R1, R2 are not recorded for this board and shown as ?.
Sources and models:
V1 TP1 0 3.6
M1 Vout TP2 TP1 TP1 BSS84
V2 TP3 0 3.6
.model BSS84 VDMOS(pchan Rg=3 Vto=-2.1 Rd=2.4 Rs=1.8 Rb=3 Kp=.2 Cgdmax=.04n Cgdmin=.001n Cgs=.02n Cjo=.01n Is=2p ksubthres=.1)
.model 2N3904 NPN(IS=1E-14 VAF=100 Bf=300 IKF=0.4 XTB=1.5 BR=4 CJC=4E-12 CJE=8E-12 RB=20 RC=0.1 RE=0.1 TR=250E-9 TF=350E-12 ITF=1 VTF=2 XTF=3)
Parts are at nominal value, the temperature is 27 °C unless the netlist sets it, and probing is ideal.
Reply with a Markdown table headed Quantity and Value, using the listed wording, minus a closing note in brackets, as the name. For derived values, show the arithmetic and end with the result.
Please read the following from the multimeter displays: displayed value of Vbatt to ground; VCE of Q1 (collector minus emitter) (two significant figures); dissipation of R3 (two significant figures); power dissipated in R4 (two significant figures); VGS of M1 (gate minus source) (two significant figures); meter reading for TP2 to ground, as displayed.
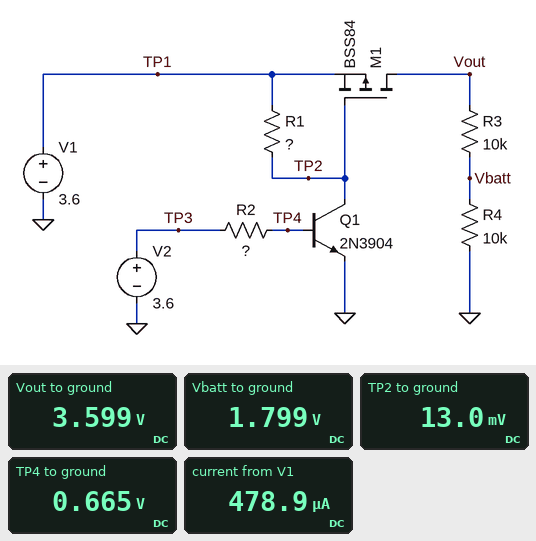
| Quantity | Value |
|---|---|
| displayed value of Vbatt to ground | 1.799 V |
| VCE of Q1 (collector minus emitter) | 13 mV = 13 mV |
| dissipation of R3 | (3.599 V - 1.799 V)^2 / 10 kΩ = 320 µW |
| power dissipated in R4 | (1.799 V)^2 / 10 kΩ = 320 µW |
| VGS of M1 (gate minus source) | 13 mV - 3.6 V = -3.6 V |
| meter reading for TP2 to ground, as displayed | 13.0 mV |
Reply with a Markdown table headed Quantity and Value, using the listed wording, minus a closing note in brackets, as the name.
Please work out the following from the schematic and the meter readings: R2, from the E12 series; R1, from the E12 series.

| Quantity | Value |
|---|---|
| R2, from the E12 series | 15 kΩ |
| R1, from the E12 series | 12 kΩ |
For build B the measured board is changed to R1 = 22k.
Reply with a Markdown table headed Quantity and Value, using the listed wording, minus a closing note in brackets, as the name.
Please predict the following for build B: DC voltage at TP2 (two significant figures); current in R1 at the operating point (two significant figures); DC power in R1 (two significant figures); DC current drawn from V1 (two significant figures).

| Quantity | Value |
|---|---|
| DC voltage at TP2 | 10 mV |
| current in R1 at the operating point | 160 µA |
| DC power in R1 | 590 µW |
| DC current drawn from V1 | 340 µA |
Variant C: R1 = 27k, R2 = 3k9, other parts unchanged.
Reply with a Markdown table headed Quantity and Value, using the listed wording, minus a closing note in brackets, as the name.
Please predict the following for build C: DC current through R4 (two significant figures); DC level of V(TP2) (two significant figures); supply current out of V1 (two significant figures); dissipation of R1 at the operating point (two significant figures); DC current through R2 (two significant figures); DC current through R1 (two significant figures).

| Quantity | Value |
|---|---|
| DC current through R4 | 180 µA |
| DC level of V(TP2) | 6.9 mV |
| supply current out of V1 | 310 µA |
| dissipation of R1 at the operating point | 480 µW |
| DC current through R2 | 740 µA |
| DC current through R1 | 130 µA |
